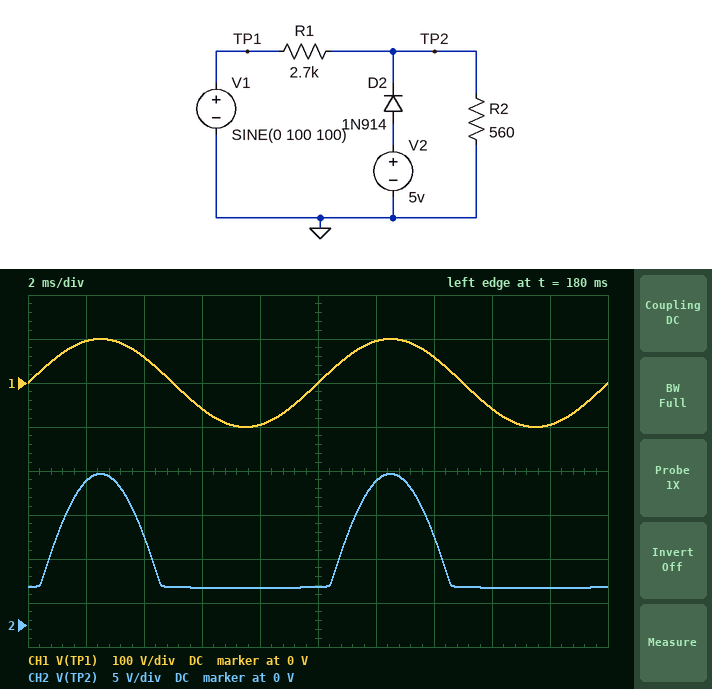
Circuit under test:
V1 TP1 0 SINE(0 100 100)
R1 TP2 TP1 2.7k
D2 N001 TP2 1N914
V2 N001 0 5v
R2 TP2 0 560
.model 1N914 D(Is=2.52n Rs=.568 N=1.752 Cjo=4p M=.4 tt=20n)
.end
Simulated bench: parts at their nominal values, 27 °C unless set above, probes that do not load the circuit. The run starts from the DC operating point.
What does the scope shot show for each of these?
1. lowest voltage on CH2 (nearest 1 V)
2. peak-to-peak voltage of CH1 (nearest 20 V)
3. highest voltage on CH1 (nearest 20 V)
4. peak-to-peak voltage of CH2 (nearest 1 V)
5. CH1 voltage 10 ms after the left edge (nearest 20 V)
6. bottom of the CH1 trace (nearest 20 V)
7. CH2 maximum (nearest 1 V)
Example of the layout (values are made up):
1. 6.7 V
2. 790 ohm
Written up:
1. 4 V
2. 200 V
3. 100 V
4. 13 V
5. 0 V
6. -100 V
7. 17 V
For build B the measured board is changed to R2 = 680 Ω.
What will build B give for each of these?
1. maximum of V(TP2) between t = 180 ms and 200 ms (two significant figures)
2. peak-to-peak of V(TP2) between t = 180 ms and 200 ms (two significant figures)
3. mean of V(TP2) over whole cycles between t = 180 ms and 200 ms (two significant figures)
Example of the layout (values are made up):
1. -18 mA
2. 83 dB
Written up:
1. 20 V
2. 16 V
3. 8.7 V
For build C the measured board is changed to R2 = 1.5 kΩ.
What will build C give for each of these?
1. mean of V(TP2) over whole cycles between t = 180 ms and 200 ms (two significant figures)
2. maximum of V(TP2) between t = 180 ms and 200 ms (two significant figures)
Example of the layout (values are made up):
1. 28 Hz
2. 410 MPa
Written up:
1. 14 V
2. 36 V
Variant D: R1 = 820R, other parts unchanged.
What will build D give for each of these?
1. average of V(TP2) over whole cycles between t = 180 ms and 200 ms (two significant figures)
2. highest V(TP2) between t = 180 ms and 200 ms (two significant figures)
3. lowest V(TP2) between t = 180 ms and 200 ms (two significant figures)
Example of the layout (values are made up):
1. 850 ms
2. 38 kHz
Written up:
1. 15 V
2. 41 V
3. 4.1 V
